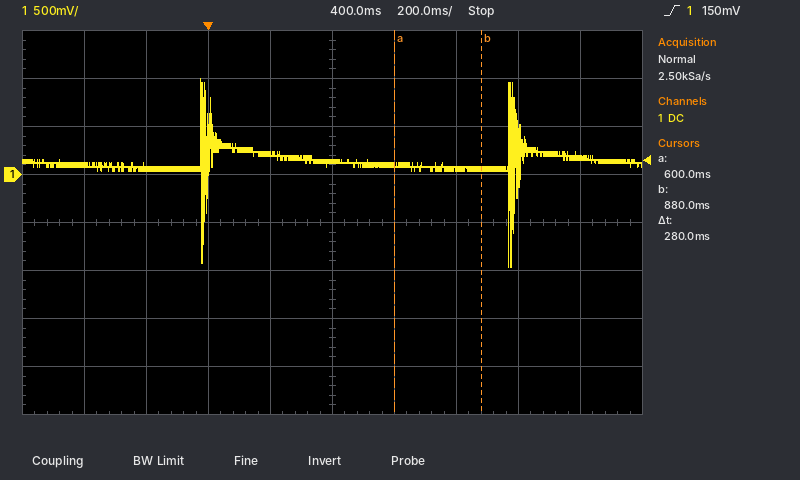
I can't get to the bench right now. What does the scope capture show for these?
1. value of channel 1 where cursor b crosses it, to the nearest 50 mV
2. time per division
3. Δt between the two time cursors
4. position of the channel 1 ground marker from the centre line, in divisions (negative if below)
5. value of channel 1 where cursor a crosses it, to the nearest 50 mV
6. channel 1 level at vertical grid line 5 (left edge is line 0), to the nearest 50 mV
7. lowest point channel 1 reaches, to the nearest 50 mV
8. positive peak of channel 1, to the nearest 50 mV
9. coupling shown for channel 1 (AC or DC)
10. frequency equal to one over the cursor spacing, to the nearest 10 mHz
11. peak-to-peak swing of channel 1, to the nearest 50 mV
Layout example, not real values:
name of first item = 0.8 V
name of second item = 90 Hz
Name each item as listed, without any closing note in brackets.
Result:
value of channel 1 where cursor b crosses it, to the nearest 50 mV = 50 mV
time per division = 200 ms
Δt between the two time cursors = 280 ms
position of the channel 1 ground marker from the centre line, in divisions = +1.0 div
value of channel 1 where cursor a crosses it, to the nearest 50 mV = 100 mV
channel 1 level at vertical grid line 5 (left edge is line 0), to the nearest 50 mV = 150 mV
lowest point channel 1 reaches, to the nearest 50 mV = -950 mV
positive peak of channel 1, to the nearest 50 mV = 1.00 V
coupling shown for channel 1 = DC
frequency equal to one over the cursor spacing, to the nearest 10 mHz = 3.57 Hz
peak-to-peak swing of channel 1, to the nearest 50 mV = 1.95 V
